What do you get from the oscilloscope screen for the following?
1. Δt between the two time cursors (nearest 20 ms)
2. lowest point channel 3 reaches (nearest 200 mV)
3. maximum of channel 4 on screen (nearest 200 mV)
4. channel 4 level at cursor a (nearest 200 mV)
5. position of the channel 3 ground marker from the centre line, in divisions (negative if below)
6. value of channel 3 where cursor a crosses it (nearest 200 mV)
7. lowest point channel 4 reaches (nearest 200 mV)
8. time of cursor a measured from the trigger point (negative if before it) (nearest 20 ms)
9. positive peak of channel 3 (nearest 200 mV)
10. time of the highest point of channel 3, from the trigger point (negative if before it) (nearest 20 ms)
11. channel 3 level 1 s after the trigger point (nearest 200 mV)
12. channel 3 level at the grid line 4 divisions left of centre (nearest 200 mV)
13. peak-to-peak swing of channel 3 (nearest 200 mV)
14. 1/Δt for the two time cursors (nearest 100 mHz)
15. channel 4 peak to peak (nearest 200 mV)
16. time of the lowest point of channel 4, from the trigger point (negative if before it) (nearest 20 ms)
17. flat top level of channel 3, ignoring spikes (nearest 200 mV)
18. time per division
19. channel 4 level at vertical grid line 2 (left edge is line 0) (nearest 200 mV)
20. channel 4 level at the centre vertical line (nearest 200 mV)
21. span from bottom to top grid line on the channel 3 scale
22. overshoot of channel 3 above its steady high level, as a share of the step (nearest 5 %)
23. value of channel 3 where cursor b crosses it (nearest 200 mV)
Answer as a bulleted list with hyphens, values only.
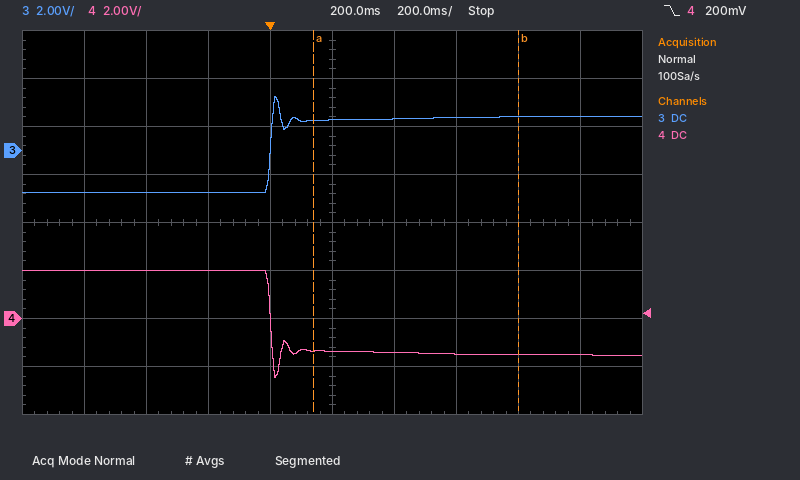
- 660 ms
- -1.8 V
- 2.0 V
- -1.4 V
- +1.5 div
- 1.2 V
- -2.4 V
- +140 ms
- 2.2 V
- +20 ms
- 1.4 V
- -1.8 V
- 4.0 V
- 1.5 Hz
- 4.4 V
- +20 ms
- 1.4 V
- 200 ms
- 2.0 V
- -1.4 V
- 16 V
- 30 %
- 1.4 V
